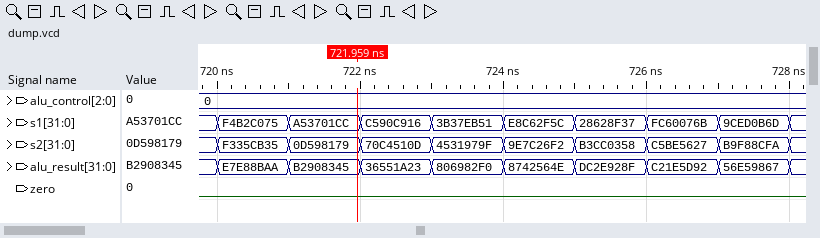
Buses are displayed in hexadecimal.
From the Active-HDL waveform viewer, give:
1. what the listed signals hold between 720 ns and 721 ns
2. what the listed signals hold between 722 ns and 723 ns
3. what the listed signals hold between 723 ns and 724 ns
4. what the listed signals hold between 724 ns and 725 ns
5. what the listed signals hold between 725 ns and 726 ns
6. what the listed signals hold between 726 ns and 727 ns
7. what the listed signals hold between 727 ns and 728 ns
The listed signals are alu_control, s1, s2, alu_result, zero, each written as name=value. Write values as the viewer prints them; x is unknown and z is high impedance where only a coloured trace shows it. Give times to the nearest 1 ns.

alu_control=0, s1=F4B2C075, s2=F335CB35, alu_result=E7E88BAA, zero=0
alu_control=0, s1=C590C916, s2=70C4510D, alu_result=36551A23, zero=0
alu_control=0, s1=3B37EB51, s2=4531979F, alu_result=806982F0, zero=0
alu_control=0, s1=E8C62F5C, s2=9E7C26F2, alu_result=8742564E, zero=0
alu_control=0, s1=28628F37, s2=B3CC0358, alu_result=DC2E928F, zero=0
alu_control=0, s1=FC60076B, s2=C5BE5627, alu_result=C21E5D92, zero=0
alu_control=0, s1=9CED0B6D, s2=B9F88CFA, alu_result=56E59867, zero=0
